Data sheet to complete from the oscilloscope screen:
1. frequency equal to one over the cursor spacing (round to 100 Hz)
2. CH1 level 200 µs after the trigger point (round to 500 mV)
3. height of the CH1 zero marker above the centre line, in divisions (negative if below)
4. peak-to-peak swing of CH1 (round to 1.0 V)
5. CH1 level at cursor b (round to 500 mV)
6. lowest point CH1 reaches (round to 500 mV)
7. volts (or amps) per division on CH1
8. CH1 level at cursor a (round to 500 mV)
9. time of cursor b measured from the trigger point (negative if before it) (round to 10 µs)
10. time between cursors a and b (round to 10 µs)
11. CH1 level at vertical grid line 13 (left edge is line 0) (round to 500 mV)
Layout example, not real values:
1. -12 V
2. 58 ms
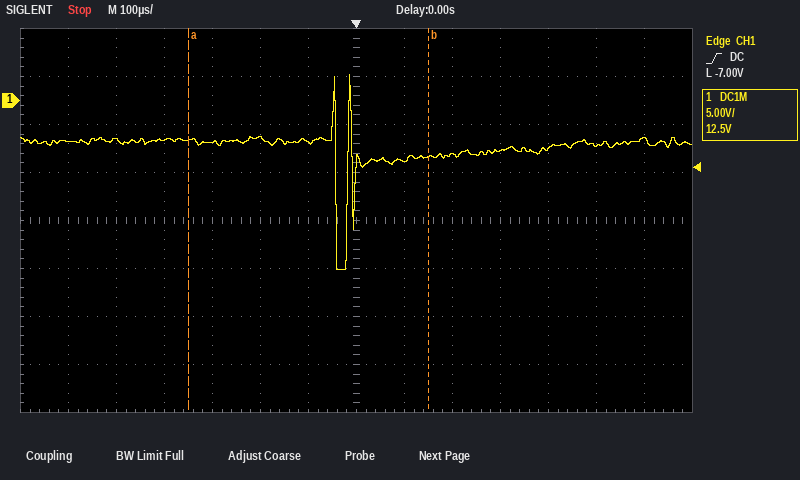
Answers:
1. 2.0 kHz
2. -5.5 V
3. +2.5 div
4. 20.0 V
5. -6.0 V
6. -17.5 V
7. 5 V
8. -4.0 V
9. +150 µs
10. 500 µs
11. -4.0 V
